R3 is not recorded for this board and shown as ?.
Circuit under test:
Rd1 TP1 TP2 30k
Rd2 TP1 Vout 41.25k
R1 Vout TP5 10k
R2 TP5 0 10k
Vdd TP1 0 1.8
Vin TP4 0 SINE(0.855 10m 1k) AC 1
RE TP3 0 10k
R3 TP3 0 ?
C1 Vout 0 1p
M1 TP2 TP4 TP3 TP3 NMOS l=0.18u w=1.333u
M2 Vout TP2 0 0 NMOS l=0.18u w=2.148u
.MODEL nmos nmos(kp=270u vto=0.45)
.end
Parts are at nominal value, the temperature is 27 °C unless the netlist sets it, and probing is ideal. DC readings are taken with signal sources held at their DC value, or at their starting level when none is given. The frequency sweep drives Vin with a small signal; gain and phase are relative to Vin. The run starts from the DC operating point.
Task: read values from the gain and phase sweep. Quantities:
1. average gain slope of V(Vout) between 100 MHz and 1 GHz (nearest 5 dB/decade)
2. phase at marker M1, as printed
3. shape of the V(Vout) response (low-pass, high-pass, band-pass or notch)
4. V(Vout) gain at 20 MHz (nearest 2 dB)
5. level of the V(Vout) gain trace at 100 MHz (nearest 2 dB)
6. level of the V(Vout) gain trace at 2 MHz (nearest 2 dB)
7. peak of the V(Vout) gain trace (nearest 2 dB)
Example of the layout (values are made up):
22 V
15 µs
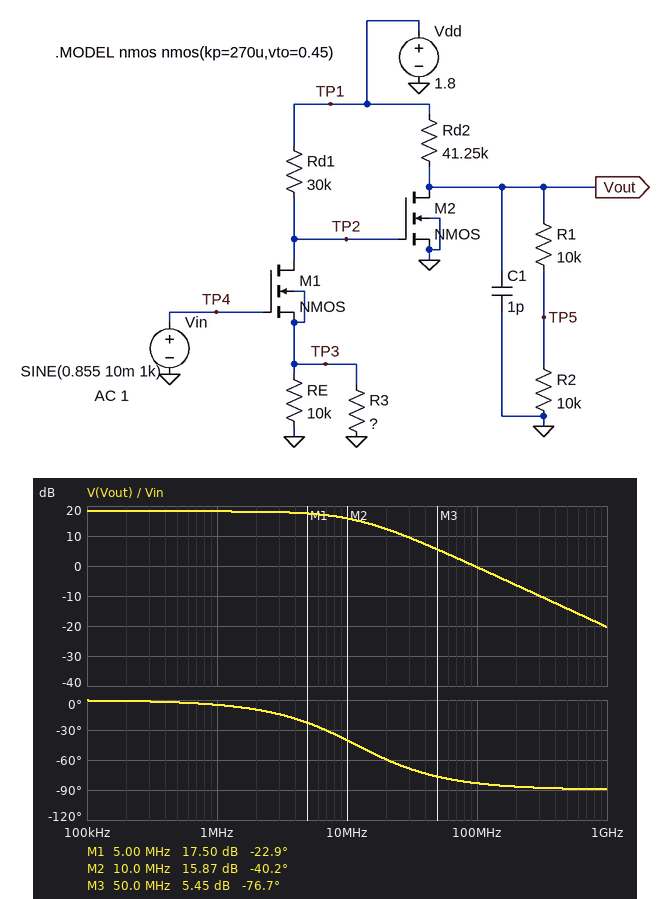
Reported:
-20 dB/decade
-22.9 deg
low-pass
12 dB
0 dB
18 dB
18 dB
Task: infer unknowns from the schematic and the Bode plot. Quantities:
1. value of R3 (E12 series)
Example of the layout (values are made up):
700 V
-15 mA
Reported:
8.2 kΩ
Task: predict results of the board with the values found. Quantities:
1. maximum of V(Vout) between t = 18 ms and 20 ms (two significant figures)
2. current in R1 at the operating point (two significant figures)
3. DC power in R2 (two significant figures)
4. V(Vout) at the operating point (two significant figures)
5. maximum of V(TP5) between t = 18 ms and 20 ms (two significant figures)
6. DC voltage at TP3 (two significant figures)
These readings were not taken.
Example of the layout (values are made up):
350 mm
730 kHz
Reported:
590 mV
27 µA
7.5 µW
550 mV
290 mV
200 mV
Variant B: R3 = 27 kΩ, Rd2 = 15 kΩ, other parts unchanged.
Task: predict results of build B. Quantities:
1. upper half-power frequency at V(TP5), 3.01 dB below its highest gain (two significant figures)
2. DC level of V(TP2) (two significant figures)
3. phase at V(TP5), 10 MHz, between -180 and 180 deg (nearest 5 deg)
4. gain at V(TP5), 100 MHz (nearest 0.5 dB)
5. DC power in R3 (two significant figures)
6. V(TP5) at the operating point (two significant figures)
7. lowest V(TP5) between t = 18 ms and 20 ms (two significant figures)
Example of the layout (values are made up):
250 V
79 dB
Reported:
180 MHz
860 mV
-5 deg
-9.5 dB
1.9 µW
46 mV
43 mV
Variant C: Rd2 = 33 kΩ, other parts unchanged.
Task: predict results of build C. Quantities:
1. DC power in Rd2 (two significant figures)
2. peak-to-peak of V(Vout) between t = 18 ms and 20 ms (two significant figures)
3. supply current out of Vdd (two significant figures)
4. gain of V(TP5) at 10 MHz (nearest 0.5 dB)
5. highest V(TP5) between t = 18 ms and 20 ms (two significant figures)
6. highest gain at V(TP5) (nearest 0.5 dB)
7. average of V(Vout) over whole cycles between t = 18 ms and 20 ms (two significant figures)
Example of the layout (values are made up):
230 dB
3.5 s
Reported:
41 µW
150 mV
79 µA
9.5 dB
340 mV
11.5 dB
620 mV
